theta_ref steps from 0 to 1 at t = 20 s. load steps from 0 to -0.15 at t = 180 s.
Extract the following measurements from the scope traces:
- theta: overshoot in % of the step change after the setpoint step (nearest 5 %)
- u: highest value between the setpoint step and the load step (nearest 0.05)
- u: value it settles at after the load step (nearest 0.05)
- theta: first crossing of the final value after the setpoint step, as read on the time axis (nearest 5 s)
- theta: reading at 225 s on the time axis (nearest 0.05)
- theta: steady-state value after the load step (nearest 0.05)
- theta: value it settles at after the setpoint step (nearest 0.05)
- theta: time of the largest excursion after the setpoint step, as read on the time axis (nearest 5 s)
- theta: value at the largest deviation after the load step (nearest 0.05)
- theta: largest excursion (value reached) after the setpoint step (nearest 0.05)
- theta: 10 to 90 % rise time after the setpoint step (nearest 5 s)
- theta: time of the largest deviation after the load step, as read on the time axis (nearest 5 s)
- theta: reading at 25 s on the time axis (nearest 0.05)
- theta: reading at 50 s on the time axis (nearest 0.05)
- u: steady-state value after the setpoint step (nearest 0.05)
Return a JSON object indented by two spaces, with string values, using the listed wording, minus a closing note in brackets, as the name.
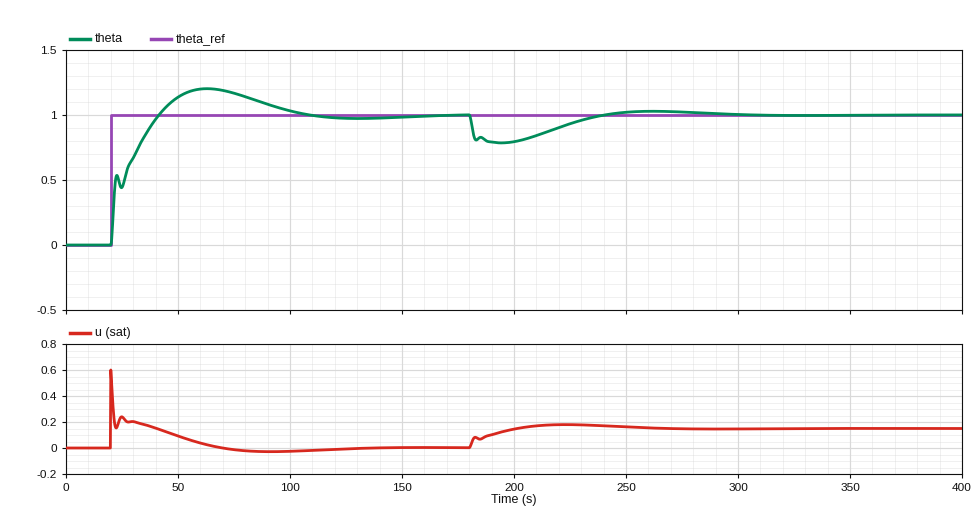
{
  "theta: overshoot in % of the step change after the setpoint step": "20 %",
  "u: highest value between the setpoint step and the load step": "0.60",
  "u: value it settles at after the load step": "0.15",
  "theta: first crossing of the final value after the setpoint step, as read on the time axis": "40 s",
  "theta: reading at 225 s on the time axis": "0.95",
  "theta: steady-state value after the load step": "1.00",
  "theta: value it settles at after the setpoint step": "1.00",
  "theta: time of the largest excursion after the setpoint step, as read on the time axis": "65 s",
  "theta: value at the largest deviation after the load step": "0.80",
  "theta: largest excursion (value reached) after the setpoint step": "1.20",
  "theta: 10 to 90 % rise time after the setpoint step": "15 s",
  "theta: time of the largest deviation after the load step, as read on the time axis": "195 s",
  "theta: reading at 25 s on the time axis": "0.45",
  "theta: reading at 50 s on the time axis": "1.15",
  "u: steady-state value after the setpoint step": "0.00"
}
